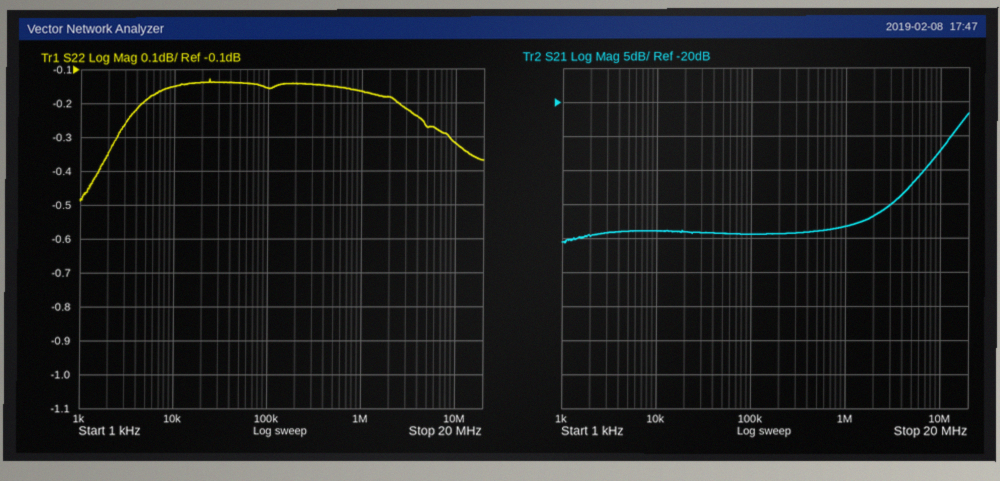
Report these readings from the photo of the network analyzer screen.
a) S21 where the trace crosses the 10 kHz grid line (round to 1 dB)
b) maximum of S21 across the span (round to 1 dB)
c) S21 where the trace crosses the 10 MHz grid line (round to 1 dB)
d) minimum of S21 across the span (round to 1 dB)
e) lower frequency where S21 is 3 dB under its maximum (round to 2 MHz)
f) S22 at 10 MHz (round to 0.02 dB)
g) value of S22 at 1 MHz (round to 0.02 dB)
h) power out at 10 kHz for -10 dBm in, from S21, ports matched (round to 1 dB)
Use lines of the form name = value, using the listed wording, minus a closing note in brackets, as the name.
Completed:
S21 where the trace crosses the 10 kHz grid line = -39 dB
maximum of S21 across the span = -22 dB
S21 where the trace crosses the 10 MHz grid line = -27 dB
minimum of S21 across the span = -41 dB
lower frequency where S21 is 3 dB under its maximum = 14 MHz
S22 at 10 MHz = -0.32 dB
value of S22 at 1 MHz = -0.16 dB
power out at 10 kHz for -10 dBm in, from S21, ports matched = -49 dBm
